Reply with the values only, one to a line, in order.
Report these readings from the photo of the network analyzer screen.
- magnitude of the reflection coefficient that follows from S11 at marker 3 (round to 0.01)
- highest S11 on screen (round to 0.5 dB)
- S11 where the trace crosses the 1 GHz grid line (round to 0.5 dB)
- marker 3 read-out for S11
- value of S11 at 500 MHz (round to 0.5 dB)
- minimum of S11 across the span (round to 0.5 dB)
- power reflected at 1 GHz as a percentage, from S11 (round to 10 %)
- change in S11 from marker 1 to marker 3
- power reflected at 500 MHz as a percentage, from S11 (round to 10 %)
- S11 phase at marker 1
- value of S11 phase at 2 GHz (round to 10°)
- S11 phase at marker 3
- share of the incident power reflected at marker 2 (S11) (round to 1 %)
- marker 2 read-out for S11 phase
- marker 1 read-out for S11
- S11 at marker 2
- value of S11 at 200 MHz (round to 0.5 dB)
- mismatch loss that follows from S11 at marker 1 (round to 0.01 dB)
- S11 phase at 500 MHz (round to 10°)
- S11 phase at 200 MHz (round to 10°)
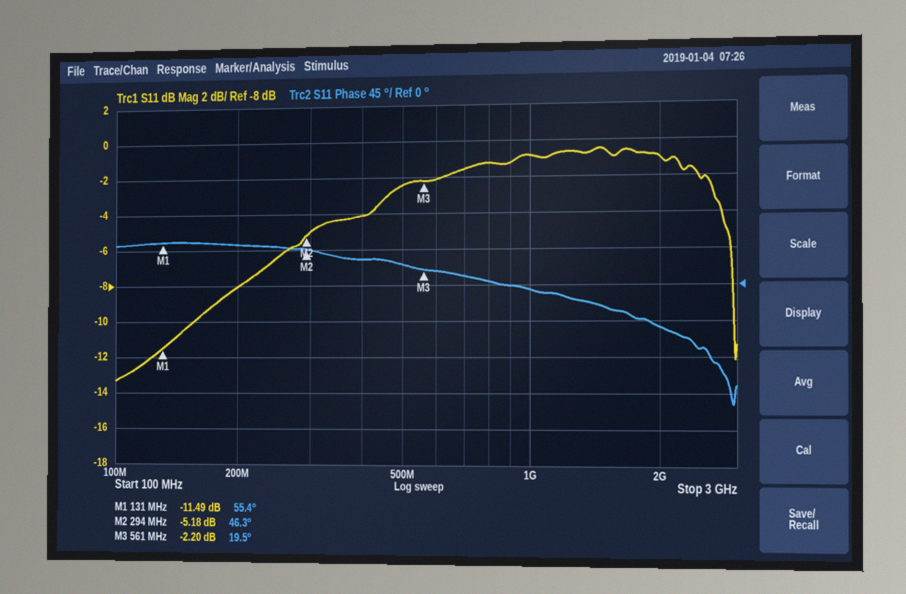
0.78
-0.5 dB
-1.0 dB
-2.20 dB
-2.5 dB
-13.5 dB
80 %
9.29 dB
60 %
55.4°
-50°
19.5°
30 %
46.3°
-11.49 dB
-5.18 dB
-8.0 dB
0.32 dB
30°
50°
